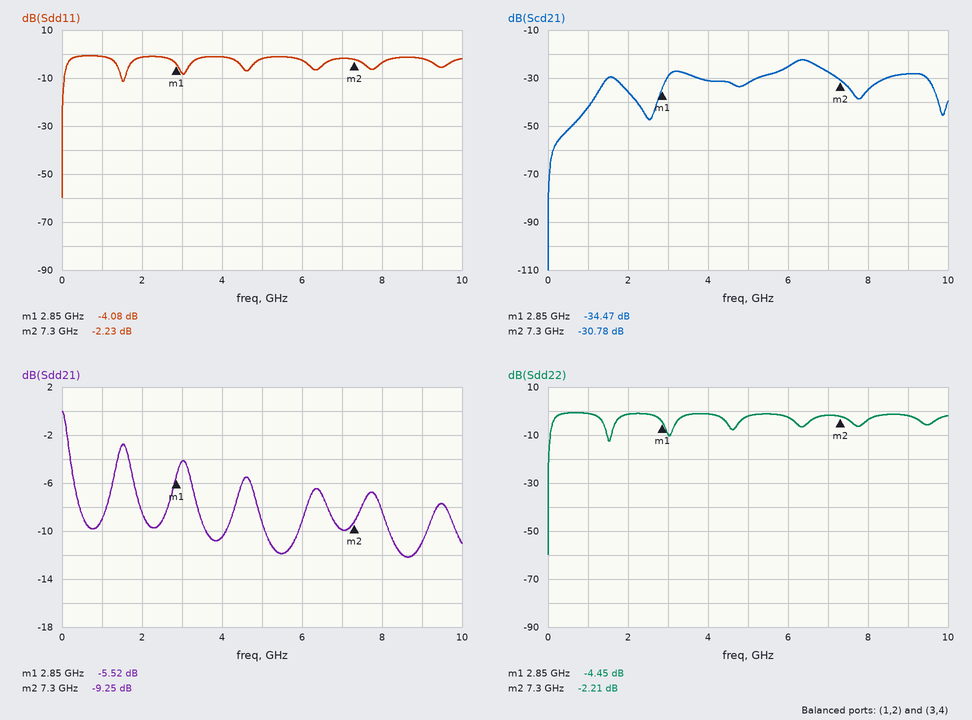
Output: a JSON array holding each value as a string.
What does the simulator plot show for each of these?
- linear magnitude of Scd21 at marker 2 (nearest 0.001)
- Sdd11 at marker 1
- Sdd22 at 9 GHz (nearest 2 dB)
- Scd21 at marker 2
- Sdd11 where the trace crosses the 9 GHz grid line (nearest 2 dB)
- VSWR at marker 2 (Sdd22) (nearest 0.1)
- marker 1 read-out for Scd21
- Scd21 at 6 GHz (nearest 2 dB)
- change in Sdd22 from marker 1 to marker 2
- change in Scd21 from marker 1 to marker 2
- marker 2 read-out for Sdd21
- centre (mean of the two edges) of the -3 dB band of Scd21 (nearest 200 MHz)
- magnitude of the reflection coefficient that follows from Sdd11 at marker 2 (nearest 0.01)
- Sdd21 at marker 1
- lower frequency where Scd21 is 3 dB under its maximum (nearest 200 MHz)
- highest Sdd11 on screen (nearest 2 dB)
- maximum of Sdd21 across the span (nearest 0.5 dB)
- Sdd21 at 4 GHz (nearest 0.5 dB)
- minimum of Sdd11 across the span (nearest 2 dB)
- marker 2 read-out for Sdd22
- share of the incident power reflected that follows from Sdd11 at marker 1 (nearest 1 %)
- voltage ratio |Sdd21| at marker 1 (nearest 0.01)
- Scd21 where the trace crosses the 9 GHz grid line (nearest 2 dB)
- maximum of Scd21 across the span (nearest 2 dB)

["0.029", "-4.08 dB", "-2 dB", "-30.78 dB", "-2 dB", "7.9", "-34.47 dB", "-26 dB", "2.24 dB", "3.69 dB", "-9.25 dB", "6.4 GHz", "0.77", "-5.52 dB", "6.0 GHz", "0 dB", "0.0 dB", "-10.5 dB", "-60 dB", "-2.21 dB", "39 %", "0.53", "-28 dB", "-22 dB"]
